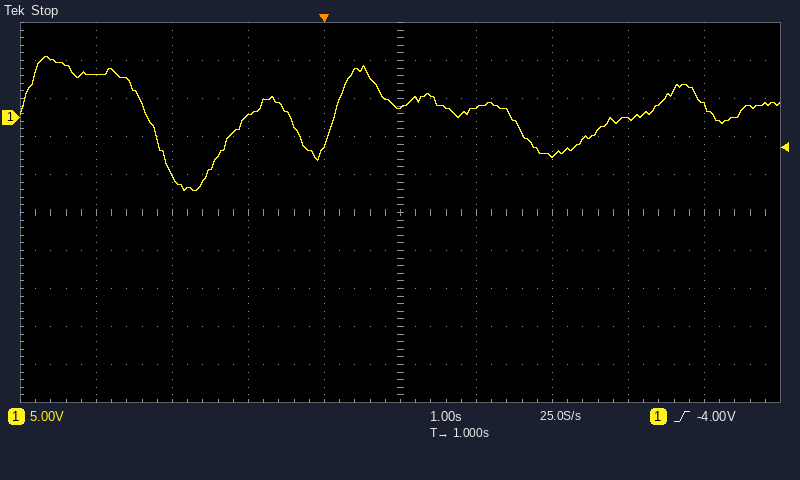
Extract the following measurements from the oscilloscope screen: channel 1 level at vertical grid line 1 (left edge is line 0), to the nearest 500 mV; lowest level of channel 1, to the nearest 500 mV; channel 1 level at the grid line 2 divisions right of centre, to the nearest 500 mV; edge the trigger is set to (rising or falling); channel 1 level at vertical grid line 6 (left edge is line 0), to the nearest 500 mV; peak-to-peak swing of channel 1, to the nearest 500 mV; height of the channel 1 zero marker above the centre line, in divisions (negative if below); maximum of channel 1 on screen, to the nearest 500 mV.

5.5 V
-9.5 V
-5.0 V
rising
1.5 V
17.5 V
+2.5 div
8.0 V
